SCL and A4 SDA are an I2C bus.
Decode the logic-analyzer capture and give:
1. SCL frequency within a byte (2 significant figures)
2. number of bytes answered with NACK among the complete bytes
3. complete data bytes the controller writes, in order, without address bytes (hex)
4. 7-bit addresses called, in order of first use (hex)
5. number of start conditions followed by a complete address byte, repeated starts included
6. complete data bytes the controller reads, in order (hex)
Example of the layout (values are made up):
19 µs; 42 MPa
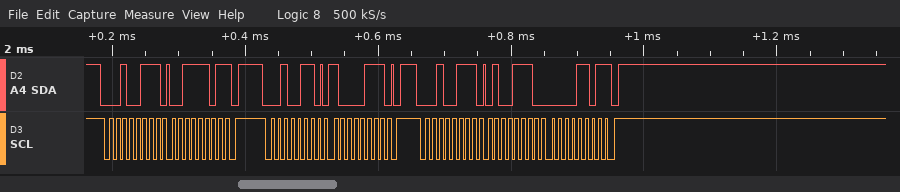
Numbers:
100 kHz; 2; 87; 0x13; 3; 3D 4E 0D
